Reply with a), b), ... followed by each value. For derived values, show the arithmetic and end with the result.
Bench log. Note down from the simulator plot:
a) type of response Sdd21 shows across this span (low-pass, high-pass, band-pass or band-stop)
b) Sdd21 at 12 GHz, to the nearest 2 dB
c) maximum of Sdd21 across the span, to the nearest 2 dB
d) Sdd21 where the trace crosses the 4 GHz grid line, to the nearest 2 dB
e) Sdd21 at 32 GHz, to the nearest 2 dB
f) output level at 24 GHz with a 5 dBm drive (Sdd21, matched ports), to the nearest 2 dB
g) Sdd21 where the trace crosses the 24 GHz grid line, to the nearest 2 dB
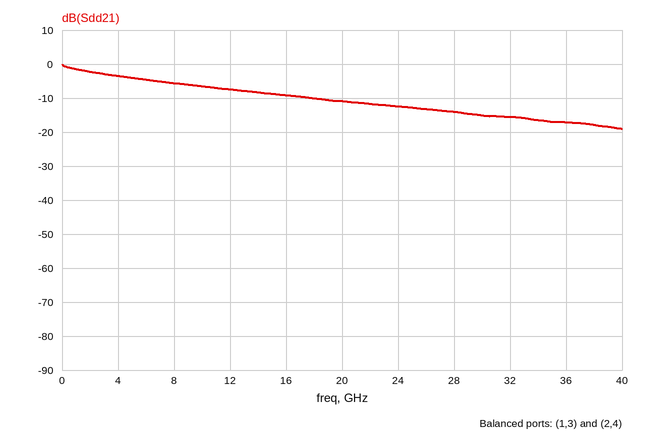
a) low-pass
b) -8 dB
c) 0 dB
d) -4 dB
e) -16 dB
f) 5 dBm + (-12 dB) = -8 dBm
g) -12 dB
